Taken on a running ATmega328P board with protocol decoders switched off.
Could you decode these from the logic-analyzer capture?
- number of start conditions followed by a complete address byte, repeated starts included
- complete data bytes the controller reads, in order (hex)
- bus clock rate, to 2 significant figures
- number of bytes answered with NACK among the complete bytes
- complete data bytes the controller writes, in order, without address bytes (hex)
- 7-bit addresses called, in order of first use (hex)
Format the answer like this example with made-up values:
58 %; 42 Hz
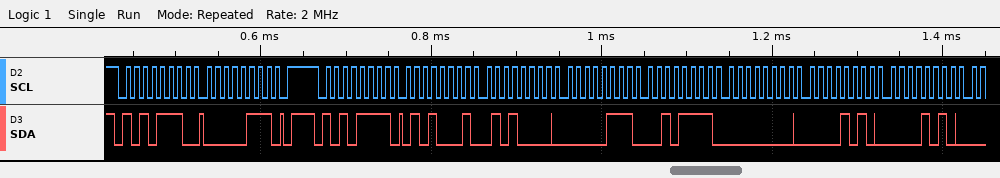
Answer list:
2; 51 50 07 2F 00 0A 0A; 100 kHz; 0; 07; 0x57
